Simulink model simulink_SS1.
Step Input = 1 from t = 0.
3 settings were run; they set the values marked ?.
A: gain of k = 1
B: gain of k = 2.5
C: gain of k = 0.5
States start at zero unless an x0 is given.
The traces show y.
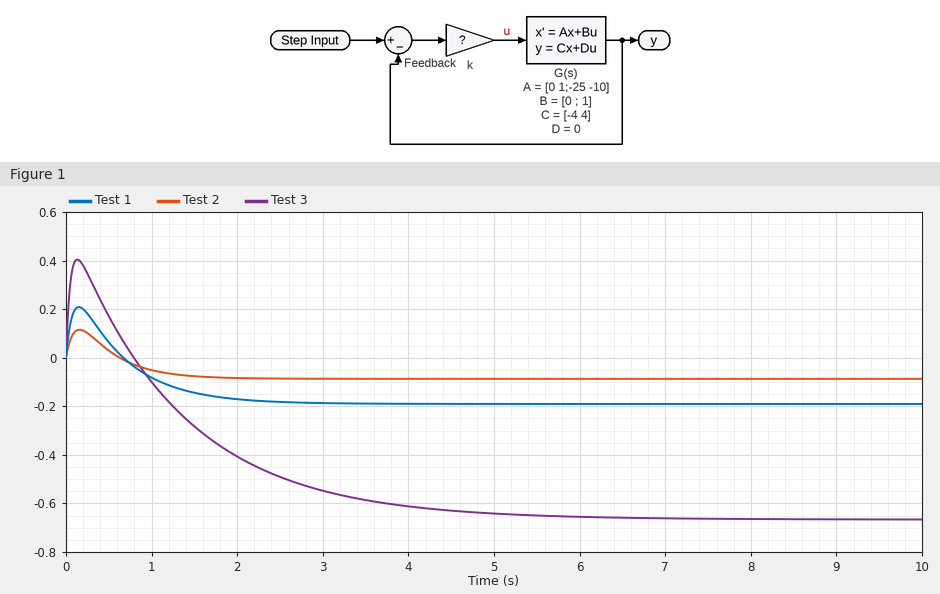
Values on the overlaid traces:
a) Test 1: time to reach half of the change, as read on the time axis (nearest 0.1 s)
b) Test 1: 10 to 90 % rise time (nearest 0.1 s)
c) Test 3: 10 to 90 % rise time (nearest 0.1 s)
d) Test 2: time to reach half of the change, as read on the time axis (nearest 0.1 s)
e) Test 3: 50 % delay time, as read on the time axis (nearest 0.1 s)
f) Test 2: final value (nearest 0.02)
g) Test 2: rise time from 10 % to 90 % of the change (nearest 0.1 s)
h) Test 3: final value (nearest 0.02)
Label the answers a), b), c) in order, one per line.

a) 1.1 s
b) 1.3 s
c) 2.8 s
d) 0.9 s
e) 1.7 s
f) -0.08
g) 0.9 s
h) -0.66
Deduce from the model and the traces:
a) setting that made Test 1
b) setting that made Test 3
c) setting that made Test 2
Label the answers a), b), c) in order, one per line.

a) A
b) B
c) C
